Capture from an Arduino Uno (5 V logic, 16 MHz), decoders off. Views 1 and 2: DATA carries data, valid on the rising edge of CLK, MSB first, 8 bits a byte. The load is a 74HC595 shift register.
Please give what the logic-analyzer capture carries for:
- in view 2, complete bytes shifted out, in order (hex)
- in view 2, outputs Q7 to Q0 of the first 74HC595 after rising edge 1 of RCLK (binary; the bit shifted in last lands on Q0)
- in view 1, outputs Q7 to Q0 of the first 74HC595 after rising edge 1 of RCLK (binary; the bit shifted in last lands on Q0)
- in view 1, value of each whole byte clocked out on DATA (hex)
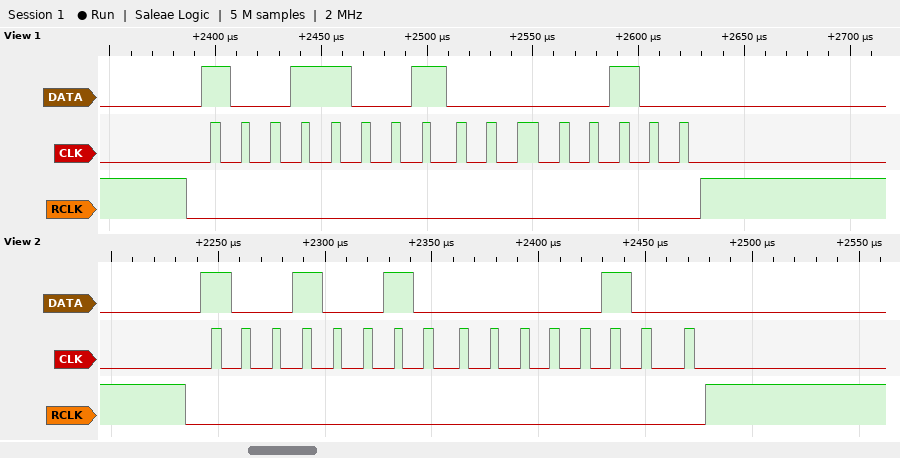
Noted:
0x92 0x04
00000100
00000100
0x99 0x04
